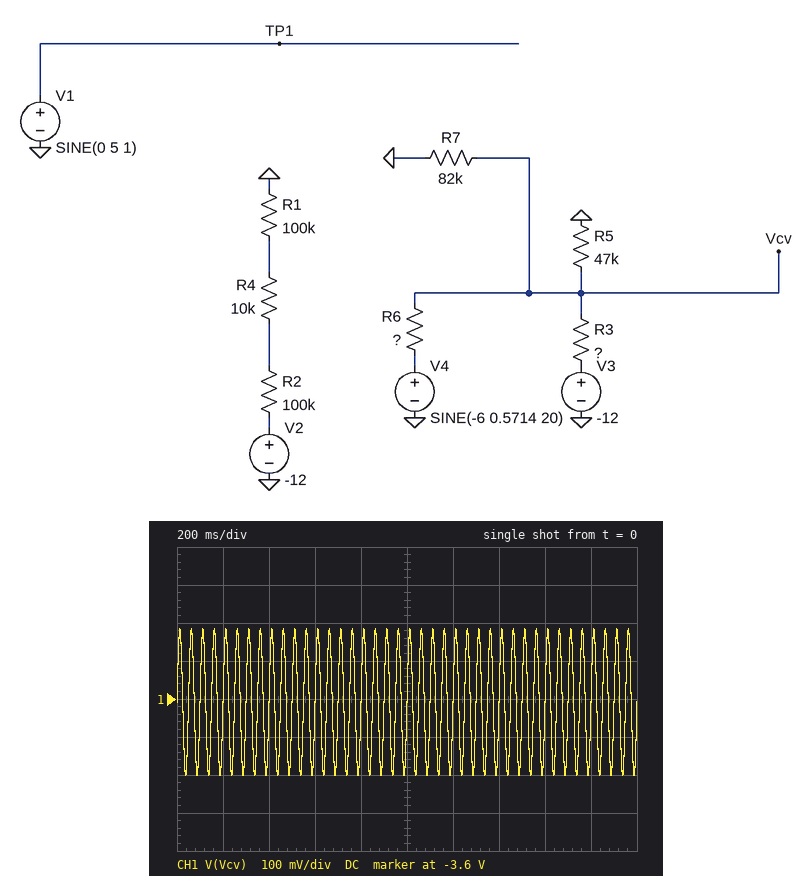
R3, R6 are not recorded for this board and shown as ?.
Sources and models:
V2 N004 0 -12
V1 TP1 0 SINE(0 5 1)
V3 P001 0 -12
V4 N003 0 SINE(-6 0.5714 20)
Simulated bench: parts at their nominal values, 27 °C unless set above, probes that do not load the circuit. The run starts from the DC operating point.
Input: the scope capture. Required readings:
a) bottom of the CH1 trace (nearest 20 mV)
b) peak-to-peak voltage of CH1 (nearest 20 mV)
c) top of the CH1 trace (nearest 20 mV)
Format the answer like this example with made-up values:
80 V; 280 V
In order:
-3.80 V; 380 mV; -3.42 V
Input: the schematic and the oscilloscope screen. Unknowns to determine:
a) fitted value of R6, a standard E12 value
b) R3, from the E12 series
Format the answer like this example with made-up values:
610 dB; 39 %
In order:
47 kΩ; 120 kΩ
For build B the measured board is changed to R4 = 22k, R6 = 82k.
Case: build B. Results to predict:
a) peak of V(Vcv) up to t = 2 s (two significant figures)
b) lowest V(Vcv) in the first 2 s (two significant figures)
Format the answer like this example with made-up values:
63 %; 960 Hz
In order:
-3.1 V; -3.3 V
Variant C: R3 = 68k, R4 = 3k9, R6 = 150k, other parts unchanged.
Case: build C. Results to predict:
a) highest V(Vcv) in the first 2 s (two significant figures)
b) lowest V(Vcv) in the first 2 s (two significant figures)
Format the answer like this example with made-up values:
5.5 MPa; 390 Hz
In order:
-3.9 V; -4.0 V
